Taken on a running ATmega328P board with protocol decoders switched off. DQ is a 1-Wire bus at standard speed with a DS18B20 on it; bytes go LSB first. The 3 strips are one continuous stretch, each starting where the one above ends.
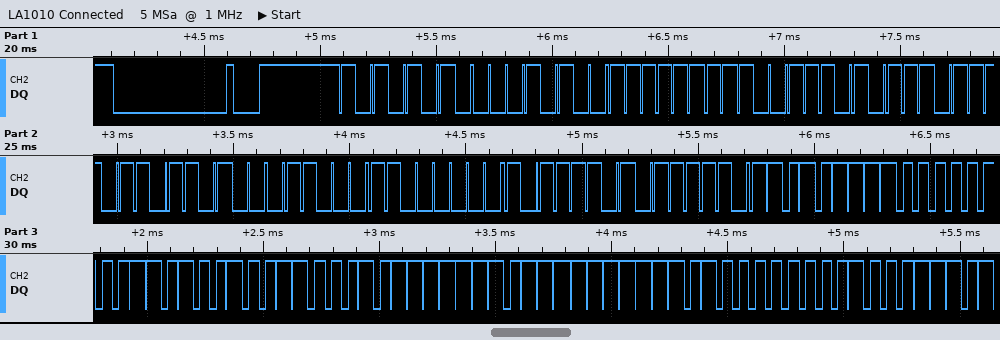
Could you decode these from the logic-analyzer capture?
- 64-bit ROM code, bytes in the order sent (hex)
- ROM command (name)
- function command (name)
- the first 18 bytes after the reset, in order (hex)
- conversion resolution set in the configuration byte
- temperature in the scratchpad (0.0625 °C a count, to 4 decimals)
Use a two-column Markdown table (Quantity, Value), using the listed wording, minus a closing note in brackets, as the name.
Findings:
| Quantity | Value |
|---|---|
| 64-bit ROM code, bytes in the order sent | 28 FF B9 EE B6 18 03 BD |
| ROM command | Match ROM |
| function command | Read Scratchpad |
| the first 18 bytes after the reset, in order | 55 28 FF B9 EE B6 18 03 BD BE F5 00 4B 46 7F FF 0B 10 |
| conversion resolution set in the configuration byte | 12 bits |
| temperature in the scratchpad | 15.3125 °C |
